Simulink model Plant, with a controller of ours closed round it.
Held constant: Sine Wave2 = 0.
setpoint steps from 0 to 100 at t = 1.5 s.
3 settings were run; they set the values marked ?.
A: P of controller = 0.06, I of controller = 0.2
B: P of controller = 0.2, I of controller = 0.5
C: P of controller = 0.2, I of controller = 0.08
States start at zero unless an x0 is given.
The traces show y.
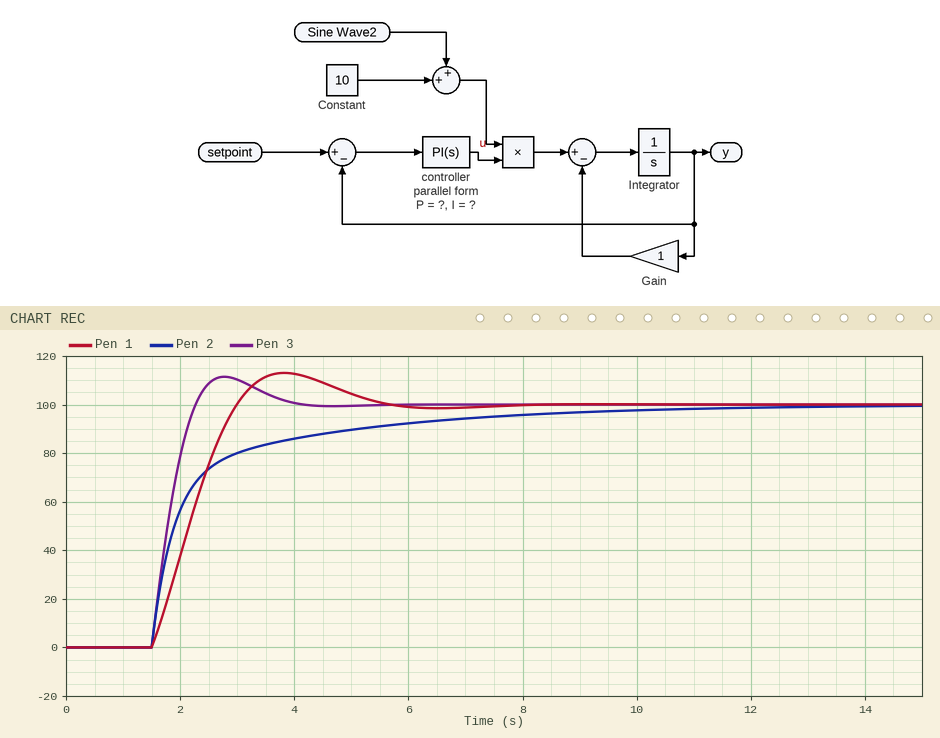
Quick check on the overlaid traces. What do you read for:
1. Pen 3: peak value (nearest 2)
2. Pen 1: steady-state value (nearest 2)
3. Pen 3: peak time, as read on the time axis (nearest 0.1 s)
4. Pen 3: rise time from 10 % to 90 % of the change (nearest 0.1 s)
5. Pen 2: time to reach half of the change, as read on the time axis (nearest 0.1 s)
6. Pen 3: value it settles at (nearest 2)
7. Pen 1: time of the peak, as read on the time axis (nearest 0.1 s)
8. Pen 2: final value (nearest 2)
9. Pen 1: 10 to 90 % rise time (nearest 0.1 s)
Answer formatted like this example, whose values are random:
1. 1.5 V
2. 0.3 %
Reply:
1. 112
2. 100
3. 2.8 s
4. 0.6 s
5. 1.9 s
6. 100
7. 3.8 s
8. 100
9. 1.1 s
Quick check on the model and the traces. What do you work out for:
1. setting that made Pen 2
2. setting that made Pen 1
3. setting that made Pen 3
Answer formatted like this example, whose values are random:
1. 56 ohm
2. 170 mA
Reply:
1. C
2. A
3. B
